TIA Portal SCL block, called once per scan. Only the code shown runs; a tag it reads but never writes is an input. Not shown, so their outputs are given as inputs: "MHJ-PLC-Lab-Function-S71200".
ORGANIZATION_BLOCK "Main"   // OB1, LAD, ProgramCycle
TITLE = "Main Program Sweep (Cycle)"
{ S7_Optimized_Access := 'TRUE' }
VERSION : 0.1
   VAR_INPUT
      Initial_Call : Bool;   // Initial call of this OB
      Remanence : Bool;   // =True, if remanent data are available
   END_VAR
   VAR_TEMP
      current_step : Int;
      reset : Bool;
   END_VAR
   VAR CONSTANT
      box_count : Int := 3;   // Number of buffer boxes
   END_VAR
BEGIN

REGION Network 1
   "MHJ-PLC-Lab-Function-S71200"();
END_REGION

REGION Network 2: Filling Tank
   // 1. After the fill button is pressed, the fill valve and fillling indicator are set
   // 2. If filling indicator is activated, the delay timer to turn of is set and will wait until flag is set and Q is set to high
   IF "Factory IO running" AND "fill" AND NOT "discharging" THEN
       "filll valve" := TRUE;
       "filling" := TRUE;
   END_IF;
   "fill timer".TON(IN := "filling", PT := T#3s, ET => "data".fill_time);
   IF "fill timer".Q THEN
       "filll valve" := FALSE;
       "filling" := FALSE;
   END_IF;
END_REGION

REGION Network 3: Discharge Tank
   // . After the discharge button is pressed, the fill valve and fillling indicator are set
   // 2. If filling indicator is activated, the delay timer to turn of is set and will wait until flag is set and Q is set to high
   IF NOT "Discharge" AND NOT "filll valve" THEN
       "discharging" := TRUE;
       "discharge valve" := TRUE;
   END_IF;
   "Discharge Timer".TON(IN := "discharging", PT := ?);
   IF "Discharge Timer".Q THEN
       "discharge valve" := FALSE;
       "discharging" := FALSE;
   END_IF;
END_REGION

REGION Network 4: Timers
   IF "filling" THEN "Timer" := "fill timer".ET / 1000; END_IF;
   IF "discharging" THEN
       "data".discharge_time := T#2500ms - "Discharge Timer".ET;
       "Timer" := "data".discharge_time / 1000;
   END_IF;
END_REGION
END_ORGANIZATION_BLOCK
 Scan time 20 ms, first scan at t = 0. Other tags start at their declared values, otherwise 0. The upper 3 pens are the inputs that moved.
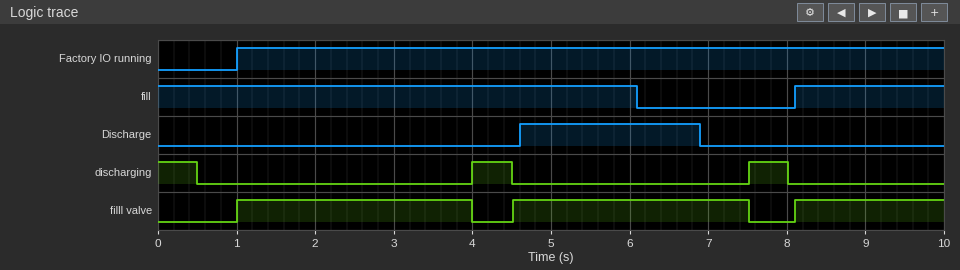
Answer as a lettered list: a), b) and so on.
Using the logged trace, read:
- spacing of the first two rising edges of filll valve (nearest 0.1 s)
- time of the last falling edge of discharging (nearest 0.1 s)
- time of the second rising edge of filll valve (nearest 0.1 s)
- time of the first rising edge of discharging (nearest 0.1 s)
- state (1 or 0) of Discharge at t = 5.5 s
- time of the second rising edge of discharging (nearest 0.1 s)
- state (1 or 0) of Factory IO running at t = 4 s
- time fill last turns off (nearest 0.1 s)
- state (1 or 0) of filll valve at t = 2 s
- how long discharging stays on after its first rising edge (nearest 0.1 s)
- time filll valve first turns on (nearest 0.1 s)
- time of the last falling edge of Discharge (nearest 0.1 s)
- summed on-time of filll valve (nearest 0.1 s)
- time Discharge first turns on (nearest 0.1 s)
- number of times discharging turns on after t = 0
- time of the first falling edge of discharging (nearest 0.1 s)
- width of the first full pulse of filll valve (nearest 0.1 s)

a) 3.5 s
b) 8.0 s
c) 4.5 s
d) 4.0 s
e) 1
f) 7.5 s
g) 1
h) 6.1 s
i) 1
j) 0.5 s
k) 1.0 s
l) 6.9 s
m) 7.9 s
n) 4.6 s
o) 2
p) 0.5 s
q) 3.0 s
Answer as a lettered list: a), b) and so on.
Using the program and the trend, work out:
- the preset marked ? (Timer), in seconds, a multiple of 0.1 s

a) 0.5 s
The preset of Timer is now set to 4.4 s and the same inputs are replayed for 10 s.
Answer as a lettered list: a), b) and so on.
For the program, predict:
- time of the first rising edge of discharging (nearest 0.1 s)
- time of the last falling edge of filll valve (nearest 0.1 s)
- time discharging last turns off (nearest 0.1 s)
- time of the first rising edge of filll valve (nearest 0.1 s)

a) 7.4 s
b) 7.4 s
c) 4.4 s
d) 4.4 s
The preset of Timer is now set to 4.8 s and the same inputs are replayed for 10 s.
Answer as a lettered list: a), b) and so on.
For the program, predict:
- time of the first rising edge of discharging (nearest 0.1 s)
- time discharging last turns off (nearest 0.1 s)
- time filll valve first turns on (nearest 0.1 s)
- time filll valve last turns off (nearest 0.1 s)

a) 7.8 s
b) 4.8 s
c) 4.8 s
d) 7.8 s
